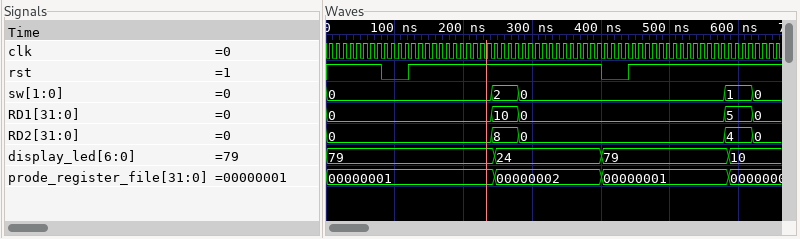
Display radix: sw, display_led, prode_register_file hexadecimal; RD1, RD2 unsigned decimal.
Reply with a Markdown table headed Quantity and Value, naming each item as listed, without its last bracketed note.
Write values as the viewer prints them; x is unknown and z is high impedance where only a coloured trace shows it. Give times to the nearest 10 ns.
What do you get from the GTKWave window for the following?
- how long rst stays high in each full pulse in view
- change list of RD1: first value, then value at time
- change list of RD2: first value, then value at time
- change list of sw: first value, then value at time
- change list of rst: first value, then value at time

| Quantity | Value |
|---|---|
| how long rst stays high in each full pulse in view | 280 ns |
| change list of RD1: first value, then value at time | 0, 10 at 240 ns, 0 at 280 ns, 5 at 580 ns, 0 at 620 ns |
| change list of RD2: first value, then value at time | 0, 8 at 240 ns, 0 at 280 ns, 4 at 580 ns, 0 at 620 ns |
| change list of sw: first value, then value at time | 0, 2 at 240 ns, 0 at 280 ns, 1 at 580 ns, 0 at 620 ns |
| change list of rst: first value, then value at time | 1, 0 at 80 ns, 1 at 120 ns, 0 at 400 ns, 1 at 440 ns |
